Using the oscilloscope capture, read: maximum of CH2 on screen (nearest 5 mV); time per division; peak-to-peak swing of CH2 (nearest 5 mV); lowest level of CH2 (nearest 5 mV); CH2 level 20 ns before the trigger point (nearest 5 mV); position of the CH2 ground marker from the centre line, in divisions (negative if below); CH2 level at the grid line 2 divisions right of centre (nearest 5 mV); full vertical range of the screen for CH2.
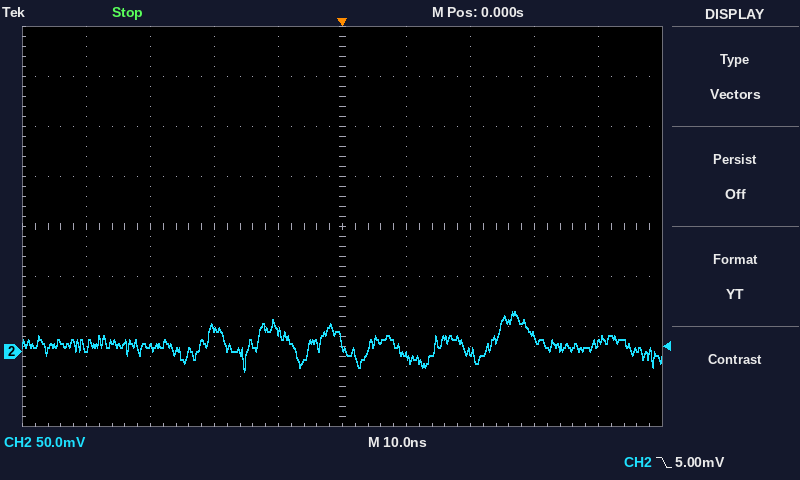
40 mV
10 ns
60 mV
-20 mV
25 mV
-2.5 div
0 mV
400 mV
